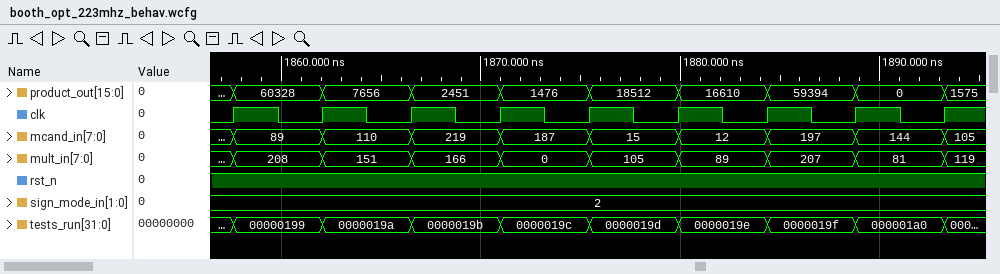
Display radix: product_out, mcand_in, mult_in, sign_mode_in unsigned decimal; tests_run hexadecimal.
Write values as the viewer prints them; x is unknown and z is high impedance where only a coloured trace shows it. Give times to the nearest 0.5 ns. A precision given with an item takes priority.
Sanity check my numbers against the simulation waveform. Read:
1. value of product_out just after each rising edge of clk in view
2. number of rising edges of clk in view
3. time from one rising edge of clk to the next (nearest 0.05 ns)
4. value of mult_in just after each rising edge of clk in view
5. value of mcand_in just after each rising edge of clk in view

60328, 7656, 2451, 1476, 18512, 16610, 59394, 0, 1575
9
4.45 ns
208, 151, 166, 0, 105, 89, 207, 81, 119
89, 110, 219, 187, 15, 12, 197, 144, 105
